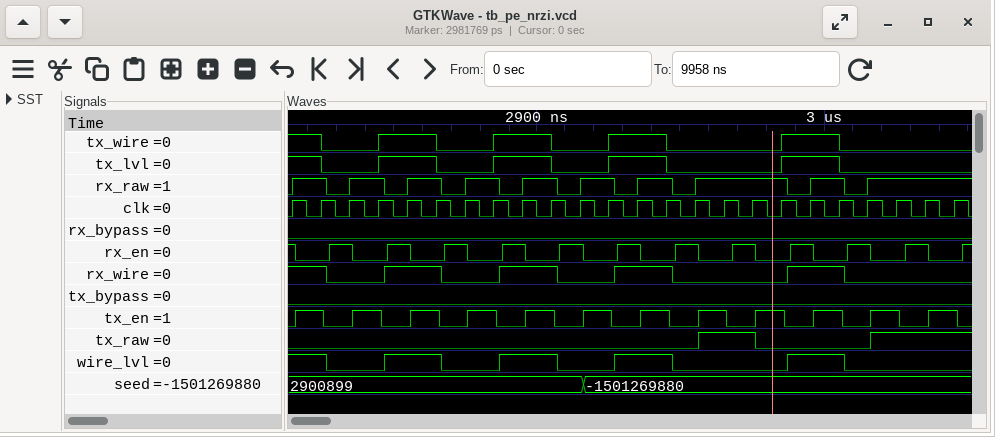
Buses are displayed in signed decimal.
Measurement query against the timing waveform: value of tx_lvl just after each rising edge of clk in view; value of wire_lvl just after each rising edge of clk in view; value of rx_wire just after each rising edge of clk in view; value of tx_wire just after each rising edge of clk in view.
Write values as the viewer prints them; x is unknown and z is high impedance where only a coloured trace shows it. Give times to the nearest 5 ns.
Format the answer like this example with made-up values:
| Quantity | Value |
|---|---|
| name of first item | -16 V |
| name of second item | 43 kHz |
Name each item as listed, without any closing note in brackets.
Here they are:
| Quantity | Value |
|---|---|
| value of tx_lvl just after each rising edge of clk in view | 1 0 0 1 1 0 0 1 1 0 0 1 1 0 0 0 0 1 1 0 0 0 0 0 |
| value of wire_lvl just after each rising edge of clk in view | 1 1 0 0 1 1 0 0 1 1 0 0 1 1 0 0 0 0 1 1 0 0 0 0 |
| value of rx_wire just after each rising edge of clk in view | 1 1 0 0 1 1 0 0 1 1 0 0 1 1 0 0 0 0 1 1 0 0 0 0 |
| value of tx_wire just after each rising edge of clk in view | 1 0 0 1 1 0 0 1 1 0 0 1 1 0 0 0 0 1 1 0 0 0 0 0 |
